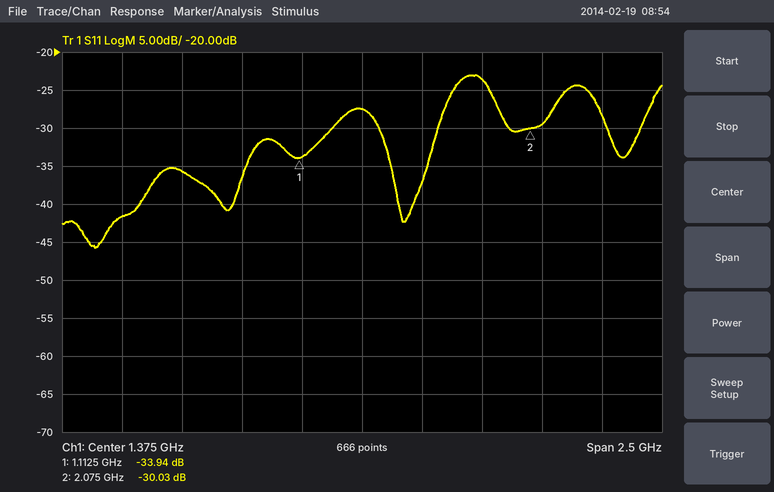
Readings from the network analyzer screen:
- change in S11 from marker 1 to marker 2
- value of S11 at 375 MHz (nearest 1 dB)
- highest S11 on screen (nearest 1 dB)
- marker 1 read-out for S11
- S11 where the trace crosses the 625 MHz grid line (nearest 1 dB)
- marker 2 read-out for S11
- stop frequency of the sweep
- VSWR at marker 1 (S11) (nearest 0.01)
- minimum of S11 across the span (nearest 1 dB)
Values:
3.91 dB
-42 dB
-23 dB
-33.94 dB
-36 dB
-30.03 dB
2.625 GHz
1.04
-46 dB
